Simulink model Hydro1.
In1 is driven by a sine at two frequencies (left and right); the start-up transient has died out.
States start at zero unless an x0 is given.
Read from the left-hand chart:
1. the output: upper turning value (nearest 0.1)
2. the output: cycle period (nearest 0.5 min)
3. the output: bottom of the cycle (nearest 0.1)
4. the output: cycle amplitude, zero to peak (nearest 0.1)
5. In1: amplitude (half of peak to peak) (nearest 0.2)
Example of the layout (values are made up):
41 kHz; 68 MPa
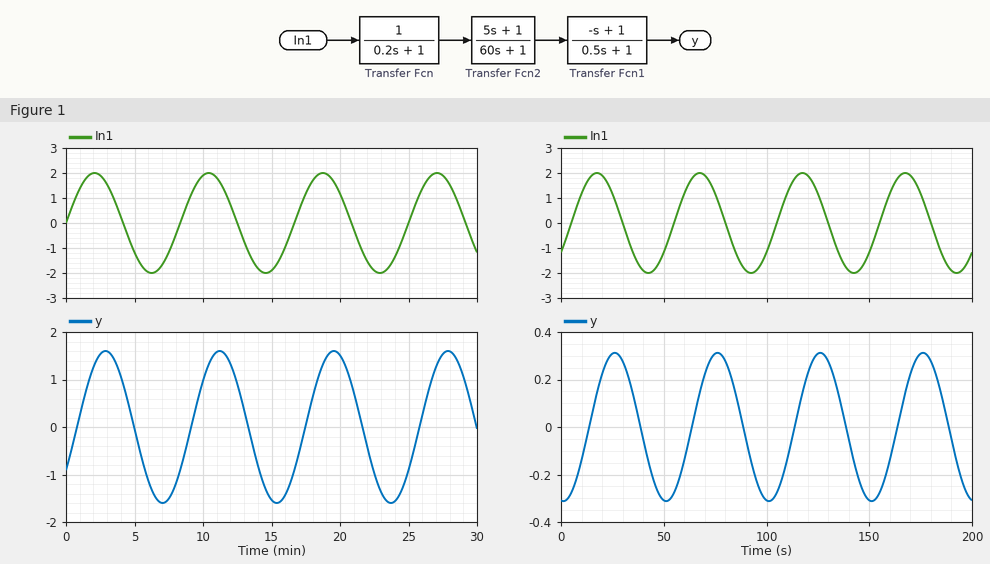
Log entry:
1.6; 8.5 min; -1.6; 1.6; 2.0
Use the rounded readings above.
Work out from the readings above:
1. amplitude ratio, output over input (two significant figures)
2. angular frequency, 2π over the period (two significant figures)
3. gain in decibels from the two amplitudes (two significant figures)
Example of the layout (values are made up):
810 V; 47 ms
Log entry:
0.80; 0.74 rad/min; -1.9 dB
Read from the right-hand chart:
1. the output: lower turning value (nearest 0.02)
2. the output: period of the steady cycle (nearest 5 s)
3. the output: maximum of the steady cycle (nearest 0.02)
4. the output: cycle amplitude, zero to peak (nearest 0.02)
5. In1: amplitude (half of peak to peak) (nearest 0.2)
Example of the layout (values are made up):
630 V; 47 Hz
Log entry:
-0.32; 50 s; 0.32; 0.32; 2.0
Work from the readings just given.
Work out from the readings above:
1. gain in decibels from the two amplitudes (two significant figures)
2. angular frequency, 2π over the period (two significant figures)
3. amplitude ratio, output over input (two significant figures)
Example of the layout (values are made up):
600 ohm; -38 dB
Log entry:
-16 dB; 0.13 rad/s; 0.16
